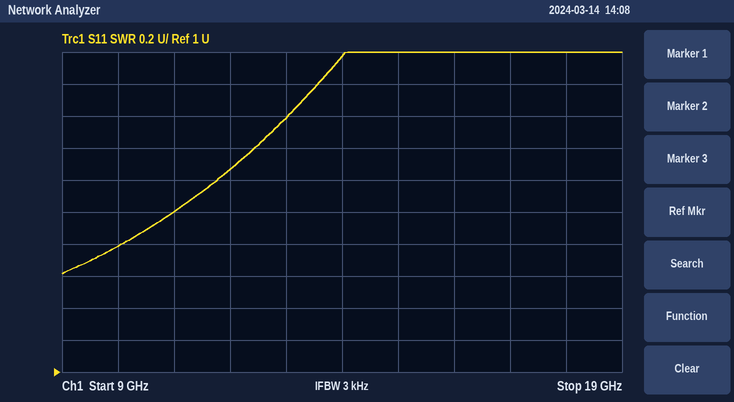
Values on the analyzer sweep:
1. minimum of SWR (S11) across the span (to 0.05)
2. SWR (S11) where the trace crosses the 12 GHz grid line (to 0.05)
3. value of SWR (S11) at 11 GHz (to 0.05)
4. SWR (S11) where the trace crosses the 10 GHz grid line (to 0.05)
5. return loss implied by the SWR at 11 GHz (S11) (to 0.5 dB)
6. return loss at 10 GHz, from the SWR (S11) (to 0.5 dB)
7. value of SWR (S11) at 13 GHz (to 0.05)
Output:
1.60
2.25
2.00
1.80
9.5 dB
11.0 dB
2.60
